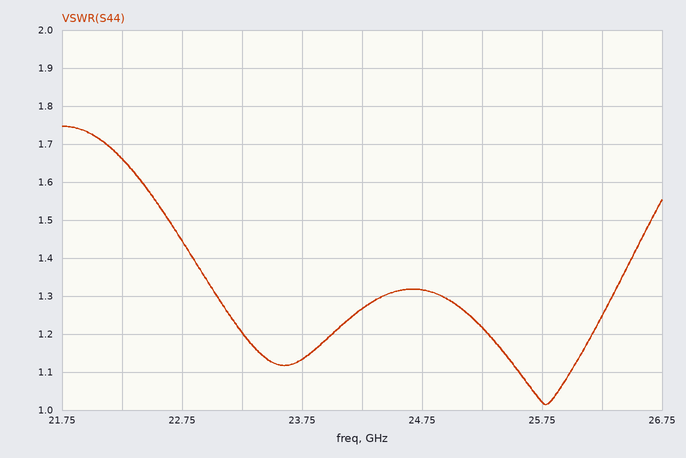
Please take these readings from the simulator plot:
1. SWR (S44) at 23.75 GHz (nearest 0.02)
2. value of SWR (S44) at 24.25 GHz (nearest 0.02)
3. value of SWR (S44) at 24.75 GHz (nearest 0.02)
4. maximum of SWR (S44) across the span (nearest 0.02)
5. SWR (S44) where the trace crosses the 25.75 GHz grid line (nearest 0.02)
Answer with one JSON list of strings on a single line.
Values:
["1.14", "1.26", "1.32", "1.74", "1.02"]
